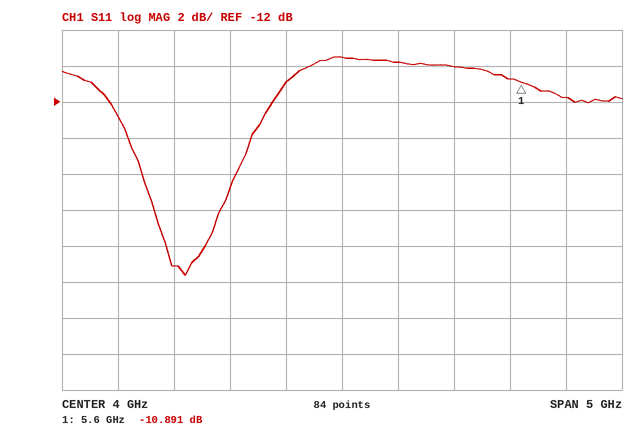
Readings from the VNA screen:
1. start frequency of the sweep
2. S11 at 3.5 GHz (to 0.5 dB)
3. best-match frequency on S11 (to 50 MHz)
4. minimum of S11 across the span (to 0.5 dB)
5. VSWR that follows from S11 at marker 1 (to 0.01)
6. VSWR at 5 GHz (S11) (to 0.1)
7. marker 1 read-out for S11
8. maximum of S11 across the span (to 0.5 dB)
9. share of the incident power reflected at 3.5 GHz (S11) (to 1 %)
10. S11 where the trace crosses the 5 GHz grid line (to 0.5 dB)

1.5 GHz
-11.0 dB
2.60 GHz
-21.5 dB
1.80
1.9
-10.891 dB
-9.5 dB
8 %
-10.0 dB
